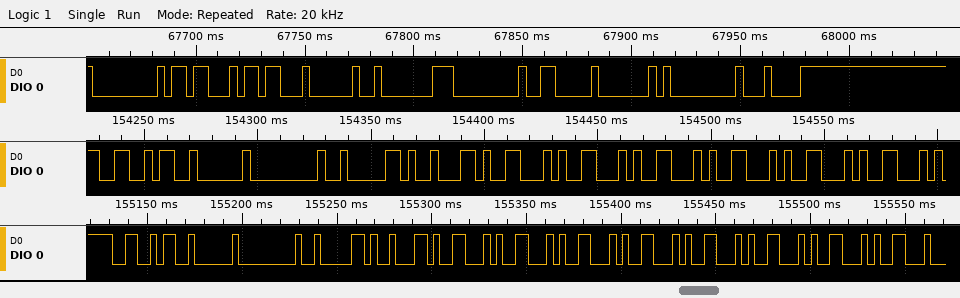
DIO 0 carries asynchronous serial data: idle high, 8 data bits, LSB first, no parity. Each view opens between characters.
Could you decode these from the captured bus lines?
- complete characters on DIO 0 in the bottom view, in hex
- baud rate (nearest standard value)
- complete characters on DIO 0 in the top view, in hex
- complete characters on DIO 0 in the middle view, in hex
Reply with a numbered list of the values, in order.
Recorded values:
1. A6, 02, 00, 82, 89, 19, 19, 19, 19, 19, 19, 19, 19
2. 300 baud
3. 00, 1B, 1B, 20, C0, 00, 06, 40, 00, 84
4. A6, 02, 00, 82, 89, 19, 19, 19, 19, 19, 19
